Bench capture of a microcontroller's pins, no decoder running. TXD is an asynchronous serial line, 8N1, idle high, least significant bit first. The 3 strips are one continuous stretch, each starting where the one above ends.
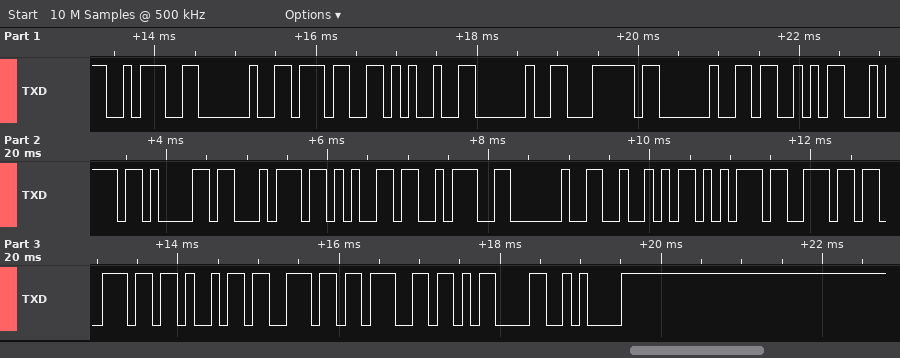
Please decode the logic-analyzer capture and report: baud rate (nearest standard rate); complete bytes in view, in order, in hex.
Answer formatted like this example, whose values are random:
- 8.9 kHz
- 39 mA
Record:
- 9600 baud
- 3A 20 37 25 20 7C 20 53 74 61 74 65 3A 20 52 75 6E 6E 69 6E 67 0D 0A
